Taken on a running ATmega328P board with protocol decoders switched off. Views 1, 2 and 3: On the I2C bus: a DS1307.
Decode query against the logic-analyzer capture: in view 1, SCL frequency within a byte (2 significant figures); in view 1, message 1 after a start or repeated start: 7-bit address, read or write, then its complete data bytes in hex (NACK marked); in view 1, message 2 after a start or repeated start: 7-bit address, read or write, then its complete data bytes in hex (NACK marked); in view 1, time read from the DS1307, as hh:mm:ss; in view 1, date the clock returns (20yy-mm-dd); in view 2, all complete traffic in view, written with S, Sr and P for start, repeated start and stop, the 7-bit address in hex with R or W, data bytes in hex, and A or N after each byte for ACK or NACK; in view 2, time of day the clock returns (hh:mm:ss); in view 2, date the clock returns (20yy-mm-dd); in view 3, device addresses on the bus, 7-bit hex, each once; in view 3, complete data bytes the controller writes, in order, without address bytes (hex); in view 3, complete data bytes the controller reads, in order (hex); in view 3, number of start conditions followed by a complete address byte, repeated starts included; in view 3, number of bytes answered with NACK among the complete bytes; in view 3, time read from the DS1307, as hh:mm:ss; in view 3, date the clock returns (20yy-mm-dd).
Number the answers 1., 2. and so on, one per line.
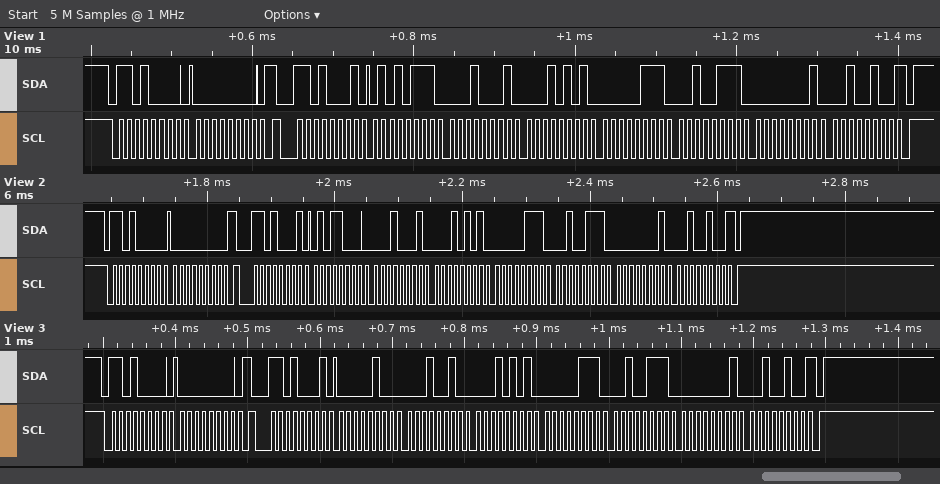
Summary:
1. 100 kHz
2. 0x68 write: 00
3. 0x68 read: 57 11 15 07 27 01 24 NACK
4. 15:11:57
5. 2024-01-27
6. S 68W A 00 A Sr 68R A 58 A 11 A 15 A 07 A 27 A 01 A 24 N P
7. 15:11:58
8. 2024-01-27
9. 0x68
10. 00
11. 04 12 15 07 27 01 24
12. 2
13. 1
14. 15:12:04
15. 2024-01-27
